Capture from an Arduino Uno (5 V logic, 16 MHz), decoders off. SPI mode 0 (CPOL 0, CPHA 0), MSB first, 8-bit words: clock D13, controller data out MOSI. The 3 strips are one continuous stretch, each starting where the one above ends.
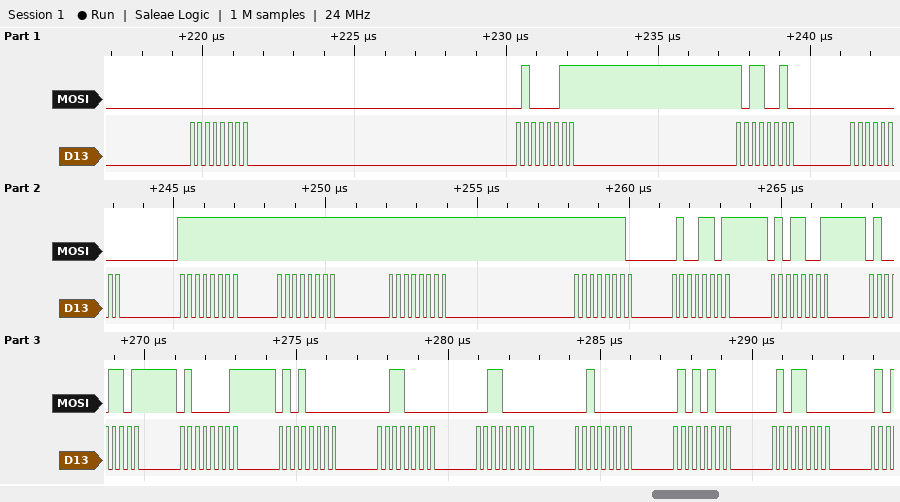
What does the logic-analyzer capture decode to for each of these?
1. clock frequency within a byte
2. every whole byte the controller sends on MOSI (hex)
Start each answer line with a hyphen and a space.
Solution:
- 4 MHz
- 00 43 B2 00 FF FF FF FE 4D 59 4D 41 50 30 30 20 54 58
